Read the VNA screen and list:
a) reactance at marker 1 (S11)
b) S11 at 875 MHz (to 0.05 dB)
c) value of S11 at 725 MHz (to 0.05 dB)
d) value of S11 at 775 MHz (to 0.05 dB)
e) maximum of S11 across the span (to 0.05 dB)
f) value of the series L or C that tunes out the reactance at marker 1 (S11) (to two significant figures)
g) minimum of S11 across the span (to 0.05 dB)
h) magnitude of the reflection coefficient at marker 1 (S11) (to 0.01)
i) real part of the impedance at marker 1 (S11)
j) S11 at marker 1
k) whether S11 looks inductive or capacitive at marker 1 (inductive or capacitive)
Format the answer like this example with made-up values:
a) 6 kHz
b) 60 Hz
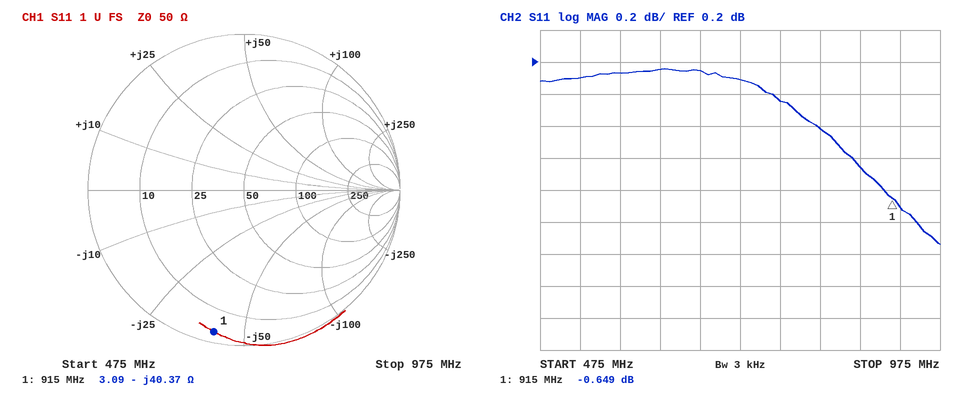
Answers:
a) -40.37 Ω
b) -0.45 dB
c) 0.10 dB
d) -0.05 dB
e) 0.15 dB
f) 7.0 nH
g) -0.95 dB
h) 0.93
i) 3.09 Ω
j) -0.649 dB
k) capacitive
